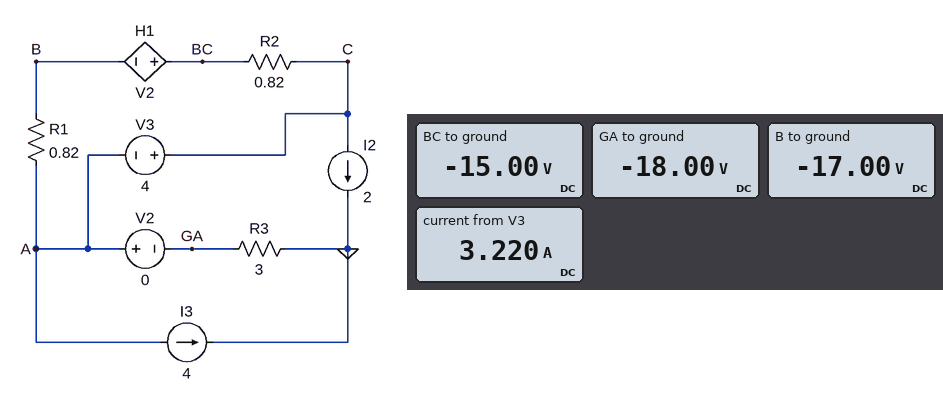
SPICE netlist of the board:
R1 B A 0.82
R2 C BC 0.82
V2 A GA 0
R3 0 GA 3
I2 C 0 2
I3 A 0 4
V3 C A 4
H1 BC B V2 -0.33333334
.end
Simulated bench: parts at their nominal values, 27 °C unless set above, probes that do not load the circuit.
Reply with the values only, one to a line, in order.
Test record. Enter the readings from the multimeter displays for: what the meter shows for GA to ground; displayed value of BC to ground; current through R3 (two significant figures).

-18.00 V
-15.00 V
6.0 A
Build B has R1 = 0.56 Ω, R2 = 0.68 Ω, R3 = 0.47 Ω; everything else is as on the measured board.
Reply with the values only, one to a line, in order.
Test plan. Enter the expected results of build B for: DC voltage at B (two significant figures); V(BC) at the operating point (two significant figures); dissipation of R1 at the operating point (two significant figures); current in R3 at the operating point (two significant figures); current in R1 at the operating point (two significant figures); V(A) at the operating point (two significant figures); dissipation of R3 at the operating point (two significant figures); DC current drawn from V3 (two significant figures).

-1.9 V
83 mV
1.5 W
6.0 A
1.6 A
-2.8 V
17 W
3.6 A
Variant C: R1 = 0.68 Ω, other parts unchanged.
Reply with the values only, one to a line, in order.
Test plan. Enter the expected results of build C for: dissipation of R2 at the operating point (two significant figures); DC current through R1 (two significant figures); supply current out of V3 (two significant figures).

1.5 W
1.3 A
3.3 A
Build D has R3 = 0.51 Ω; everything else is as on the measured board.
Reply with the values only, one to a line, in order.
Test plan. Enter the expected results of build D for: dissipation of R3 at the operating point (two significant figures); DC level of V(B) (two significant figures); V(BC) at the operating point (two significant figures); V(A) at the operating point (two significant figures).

18 W
-2.1 V
-60 mV
-3.1 V
